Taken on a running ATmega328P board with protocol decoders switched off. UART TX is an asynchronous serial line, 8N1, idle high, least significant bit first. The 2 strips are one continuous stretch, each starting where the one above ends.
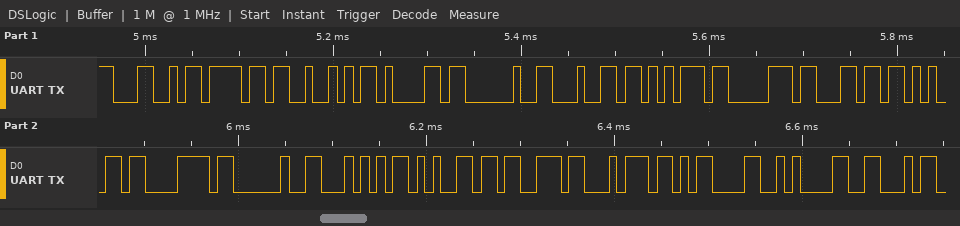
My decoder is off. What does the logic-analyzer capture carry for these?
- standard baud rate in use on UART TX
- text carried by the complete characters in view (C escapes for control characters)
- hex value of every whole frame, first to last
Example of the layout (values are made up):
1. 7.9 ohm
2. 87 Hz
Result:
1. 115200 baud
2. "LoRa duplex Test\r\nF"
3. 4C 6F 52 61 20 64 75 70 6C 65 78 20 54 65 73 74 0D 0A 46
